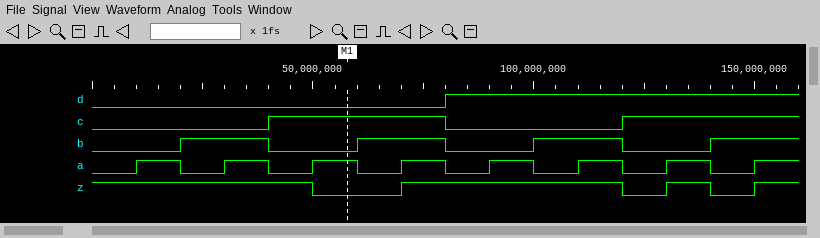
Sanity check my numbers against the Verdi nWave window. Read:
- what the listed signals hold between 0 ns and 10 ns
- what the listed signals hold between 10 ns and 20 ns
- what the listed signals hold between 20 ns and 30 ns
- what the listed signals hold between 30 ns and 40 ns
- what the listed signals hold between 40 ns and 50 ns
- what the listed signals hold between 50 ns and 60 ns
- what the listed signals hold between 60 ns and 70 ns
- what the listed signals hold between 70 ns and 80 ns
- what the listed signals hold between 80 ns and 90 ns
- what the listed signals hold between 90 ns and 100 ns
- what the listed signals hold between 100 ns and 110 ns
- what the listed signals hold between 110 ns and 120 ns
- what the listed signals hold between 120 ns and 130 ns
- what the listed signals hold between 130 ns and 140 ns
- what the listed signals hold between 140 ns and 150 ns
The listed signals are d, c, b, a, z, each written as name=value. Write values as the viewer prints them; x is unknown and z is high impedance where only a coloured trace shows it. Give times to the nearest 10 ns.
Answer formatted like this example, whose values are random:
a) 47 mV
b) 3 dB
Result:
a) d=0, c=0, b=0, a=0, z=1
b) d=0, c=0, b=0, a=1, z=1
c) d=0, c=0, b=1, a=0, z=1
d) d=0, c=0, b=1, a=1, z=1
e) d=0, c=1, b=0, a=0, z=1
f) d=0, c=1, b=0, a=1, z=0
g) d=0, c=1, b=1, a=0, z=0
h) d=0, c=1, b=1, a=1, z=1
i) d=1, c=0, b=0, a=0, z=1
j) d=1, c=0, b=0, a=1, z=1
k) d=1, c=0, b=1, a=0, z=1
l) d=1, c=0, b=1, a=1, z=1
m) d=1, c=1, b=0, a=0, z=0
n) d=1, c=1, b=0, a=1, z=1
o) d=1, c=1, b=1, a=0, z=0
